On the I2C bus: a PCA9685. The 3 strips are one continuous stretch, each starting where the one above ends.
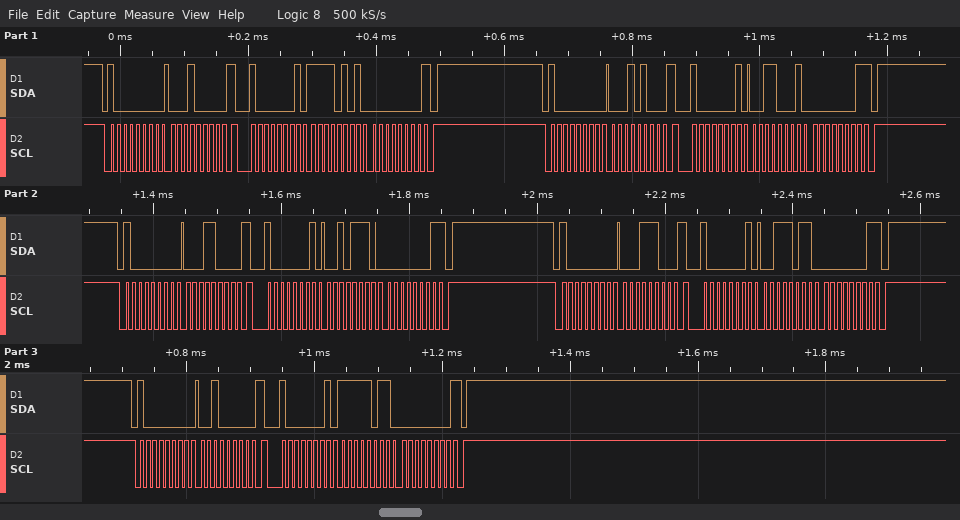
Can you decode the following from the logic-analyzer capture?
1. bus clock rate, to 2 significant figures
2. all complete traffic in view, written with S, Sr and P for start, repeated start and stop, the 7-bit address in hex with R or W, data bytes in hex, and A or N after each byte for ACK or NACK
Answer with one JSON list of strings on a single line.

["100 kHz", "S 40W A 10 A Sr 40R A F5 A 00 N P S 40W A 14 A Sr 40R A 31 A 01 N P S 40W A 18 A Sr 40R A 2E A 01 N P S 40W A 1C A Sr 40R A 3B A 01 N P S 40W A 20 A Sr 40R A FB A 00 N P"]
